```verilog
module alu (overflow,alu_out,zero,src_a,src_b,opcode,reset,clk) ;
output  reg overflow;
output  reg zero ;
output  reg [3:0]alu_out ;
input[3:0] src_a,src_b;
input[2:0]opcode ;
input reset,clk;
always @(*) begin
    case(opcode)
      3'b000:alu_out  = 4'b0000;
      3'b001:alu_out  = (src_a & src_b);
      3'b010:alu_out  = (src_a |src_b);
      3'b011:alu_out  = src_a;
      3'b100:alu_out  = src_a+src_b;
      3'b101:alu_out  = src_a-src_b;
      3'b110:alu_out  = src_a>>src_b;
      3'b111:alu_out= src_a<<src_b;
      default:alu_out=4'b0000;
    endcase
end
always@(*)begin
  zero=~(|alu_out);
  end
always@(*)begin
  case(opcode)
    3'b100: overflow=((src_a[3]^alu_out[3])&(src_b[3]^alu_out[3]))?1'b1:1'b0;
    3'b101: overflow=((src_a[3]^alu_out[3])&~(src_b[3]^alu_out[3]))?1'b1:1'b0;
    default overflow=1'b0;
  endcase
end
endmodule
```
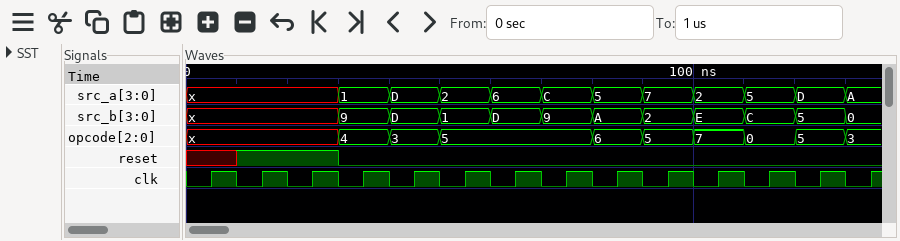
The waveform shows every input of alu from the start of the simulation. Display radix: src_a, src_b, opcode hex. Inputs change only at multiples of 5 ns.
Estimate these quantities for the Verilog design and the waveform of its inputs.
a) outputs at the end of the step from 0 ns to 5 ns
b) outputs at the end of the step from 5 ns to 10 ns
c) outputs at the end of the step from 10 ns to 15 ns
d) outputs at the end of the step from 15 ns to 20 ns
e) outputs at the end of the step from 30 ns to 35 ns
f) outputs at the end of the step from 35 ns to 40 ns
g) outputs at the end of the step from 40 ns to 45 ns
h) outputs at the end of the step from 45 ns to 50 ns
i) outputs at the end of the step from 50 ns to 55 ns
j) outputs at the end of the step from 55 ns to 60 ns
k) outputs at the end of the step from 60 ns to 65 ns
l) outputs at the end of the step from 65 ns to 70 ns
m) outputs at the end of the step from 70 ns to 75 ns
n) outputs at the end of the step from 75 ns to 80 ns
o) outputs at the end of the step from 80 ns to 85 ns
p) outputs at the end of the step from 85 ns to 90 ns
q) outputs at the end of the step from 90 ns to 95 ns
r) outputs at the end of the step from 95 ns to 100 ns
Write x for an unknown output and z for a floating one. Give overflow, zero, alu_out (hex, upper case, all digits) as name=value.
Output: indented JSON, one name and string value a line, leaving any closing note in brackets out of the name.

{
  "outputs at the end of the step from 0 ns to 5 ns": "overflow=x, zero=x, alu_out=x",
  "outputs at the end of the step from 5 ns to 10 ns": "overflow=x, zero=x, alu_out=x",
  "outputs at the end of the step from 10 ns to 15 ns": "overflow=x, zero=x, alu_out=x",
  "outputs at the end of the step from 15 ns to 20 ns": "overflow=x, zero=x, alu_out=x",
  "outputs at the end of the step from 30 ns to 35 ns": "overflow=0, zero=0, alu_out=A",
  "outputs at the end of the step from 35 ns to 40 ns": "overflow=0, zero=0, alu_out=A",
  "outputs at the end of the step from 40 ns to 45 ns": "overflow=0, zero=0, alu_out=D",
  "outputs at the end of the step from 45 ns to 50 ns": "overflow=0, zero=0, alu_out=D",
  "outputs at the end of the step from 50 ns to 55 ns": "overflow=0, zero=0, alu_out=1",
  "outputs at the end of the step from 55 ns to 60 ns": "overflow=0, zero=0, alu_out=1",
  "outputs at the end of the step from 60 ns to 65 ns": "overflow=1, zero=0, alu_out=9",
  "outputs at the end of the step from 65 ns to 70 ns": "overflow=1, zero=0, alu_out=9",
  "outputs at the end of the step from 70 ns to 75 ns": "overflow=0, zero=0, alu_out=3",
  "outputs at the end of the step from 75 ns to 80 ns": "overflow=0, zero=0, alu_out=3",
  "outputs at the end of the step from 80 ns to 85 ns": "overflow=0, zero=1, alu_out=0",
  "outputs at the end of the step from 85 ns to 90 ns": "overflow=0, zero=1, alu_out=0",
  "outputs at the end of the step from 90 ns to 95 ns": "overflow=0, zero=0, alu_out=5",
  "outputs at the end of the step from 95 ns to 100 ns": "overflow=0, zero=0, alu_out=5"
}
